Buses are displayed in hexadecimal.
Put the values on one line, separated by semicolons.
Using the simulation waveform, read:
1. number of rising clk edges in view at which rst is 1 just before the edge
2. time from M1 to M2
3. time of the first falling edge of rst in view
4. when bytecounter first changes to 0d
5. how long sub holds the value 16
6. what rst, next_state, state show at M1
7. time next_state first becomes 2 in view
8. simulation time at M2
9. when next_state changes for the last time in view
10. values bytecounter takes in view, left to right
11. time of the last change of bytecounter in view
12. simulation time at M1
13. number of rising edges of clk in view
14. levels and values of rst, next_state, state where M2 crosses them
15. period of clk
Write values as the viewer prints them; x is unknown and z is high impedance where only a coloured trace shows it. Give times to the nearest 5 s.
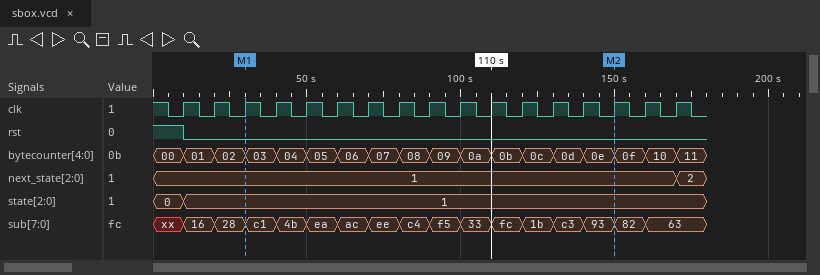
1; 120 s; 10 s; 130 s; 10 s; rst=0, next_state=1, state=1; 170 s; 150 s; 170 s; 00, 01, 02, 03, 04, 05, 06, 07, 08, 09, 0a, 0b, 0c, 0d, 0e, 0f, 10, 11; 170 s; 30 s; 17; rst=0, next_state=1, state=1; 10 s
